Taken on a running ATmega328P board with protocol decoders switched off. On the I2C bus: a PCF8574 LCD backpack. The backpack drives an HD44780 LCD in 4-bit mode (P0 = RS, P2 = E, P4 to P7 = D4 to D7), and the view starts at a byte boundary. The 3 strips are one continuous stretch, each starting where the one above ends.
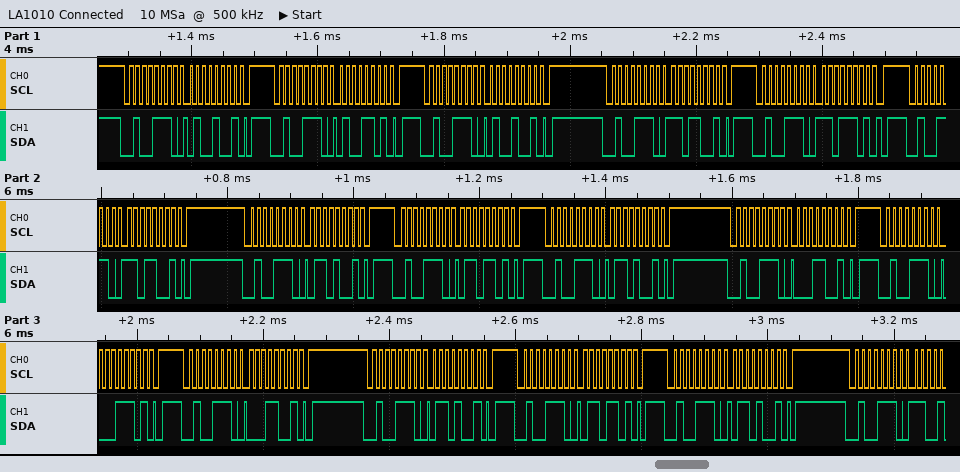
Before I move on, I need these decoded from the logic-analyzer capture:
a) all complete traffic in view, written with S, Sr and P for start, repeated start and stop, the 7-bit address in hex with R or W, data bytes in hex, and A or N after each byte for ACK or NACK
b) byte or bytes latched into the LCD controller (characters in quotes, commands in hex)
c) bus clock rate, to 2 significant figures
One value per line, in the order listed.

S 27W A 49 A P S 27W A 4D A P S 27W A 49 A P S 27W A D9 A P S 27W A DD A P S 27W A D9 A P S 27W A 69 A P S 27W A 6D A P S 27W A 69 A P S 27W A 19 A P S 27W A 1D A P S 27W A 19 A P S 27W A 69 A P S 27W A 6D A P S 27W A 69 A P S 27W A
'M' 'a'
100 kHz
